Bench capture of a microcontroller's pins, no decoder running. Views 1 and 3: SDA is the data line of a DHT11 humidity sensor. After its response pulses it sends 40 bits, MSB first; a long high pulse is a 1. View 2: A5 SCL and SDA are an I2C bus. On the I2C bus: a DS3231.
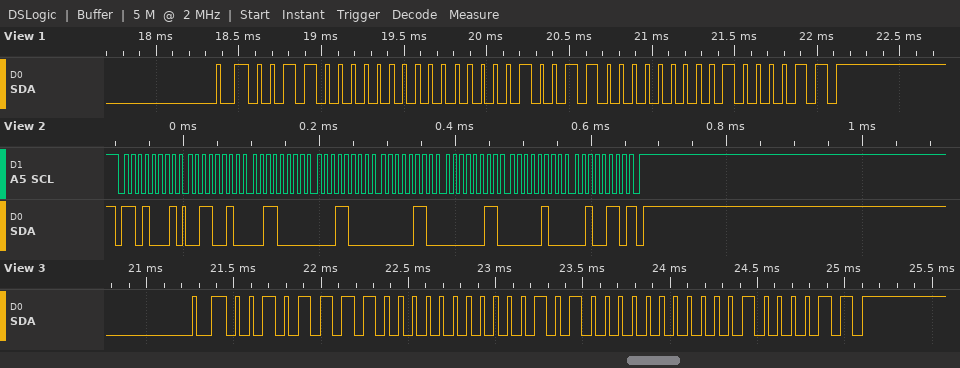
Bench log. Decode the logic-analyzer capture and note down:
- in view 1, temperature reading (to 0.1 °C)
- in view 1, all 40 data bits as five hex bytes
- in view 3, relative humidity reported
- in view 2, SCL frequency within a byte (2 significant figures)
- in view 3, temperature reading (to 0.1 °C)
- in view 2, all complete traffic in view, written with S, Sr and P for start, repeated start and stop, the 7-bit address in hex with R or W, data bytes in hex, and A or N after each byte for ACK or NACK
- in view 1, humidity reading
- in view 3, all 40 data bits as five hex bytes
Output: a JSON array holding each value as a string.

["19.0 °C", "30 00 13 00 43", "47 %", "100 kHz", "20.0 °C", "S 68R A 32 A 30 A 18 A 06 A 03 A 04 A 26 N P", "48 %", "2F 00 14 00 43"]
